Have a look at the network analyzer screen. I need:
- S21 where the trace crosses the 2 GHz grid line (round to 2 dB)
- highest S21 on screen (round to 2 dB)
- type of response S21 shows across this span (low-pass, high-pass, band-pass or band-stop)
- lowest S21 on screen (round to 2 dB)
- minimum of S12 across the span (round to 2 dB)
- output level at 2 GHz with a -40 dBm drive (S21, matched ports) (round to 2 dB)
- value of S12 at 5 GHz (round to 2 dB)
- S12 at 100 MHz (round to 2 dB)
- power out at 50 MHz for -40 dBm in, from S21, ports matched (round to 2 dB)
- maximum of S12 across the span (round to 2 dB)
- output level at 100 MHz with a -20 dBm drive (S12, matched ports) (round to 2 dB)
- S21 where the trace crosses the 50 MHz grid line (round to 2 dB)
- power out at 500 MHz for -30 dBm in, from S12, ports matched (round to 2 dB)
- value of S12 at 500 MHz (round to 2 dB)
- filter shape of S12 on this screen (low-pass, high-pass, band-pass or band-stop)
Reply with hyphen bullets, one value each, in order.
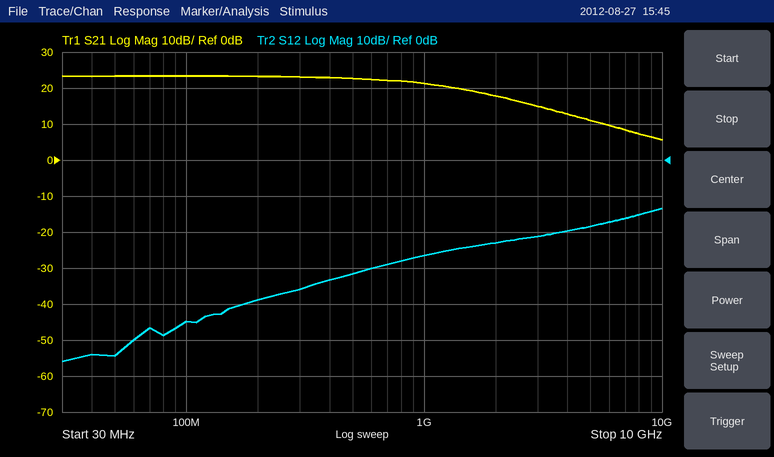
- 18 dB
- 24 dB
- low-pass
- 6 dB
- -56 dB
- -22 dBm
- -18 dB
- -44 dB
- -16 dBm
- -14 dB
- -64 dBm
- 24 dB
- -62 dBm
- -32 dB
- high-pass
